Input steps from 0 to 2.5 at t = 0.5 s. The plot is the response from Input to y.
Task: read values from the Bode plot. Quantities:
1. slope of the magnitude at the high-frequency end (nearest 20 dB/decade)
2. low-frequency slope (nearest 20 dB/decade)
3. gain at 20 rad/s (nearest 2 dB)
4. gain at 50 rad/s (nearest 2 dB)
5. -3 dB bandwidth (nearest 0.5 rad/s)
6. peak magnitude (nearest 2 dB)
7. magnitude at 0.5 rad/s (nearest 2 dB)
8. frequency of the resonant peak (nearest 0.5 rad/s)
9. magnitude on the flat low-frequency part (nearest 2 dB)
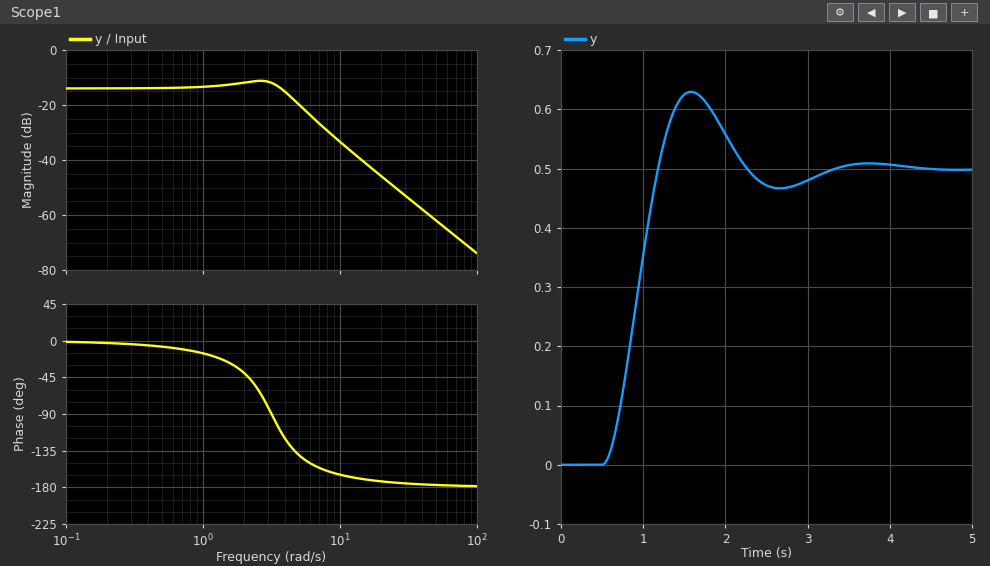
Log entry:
-40 dB/decade
0 dB/decade
-46 dB
-62 dB
4.5 rad/s
-12 dB
-14 dB
2.5 rad/s
-14 dB
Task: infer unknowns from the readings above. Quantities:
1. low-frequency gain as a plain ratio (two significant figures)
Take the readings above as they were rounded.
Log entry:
0.20
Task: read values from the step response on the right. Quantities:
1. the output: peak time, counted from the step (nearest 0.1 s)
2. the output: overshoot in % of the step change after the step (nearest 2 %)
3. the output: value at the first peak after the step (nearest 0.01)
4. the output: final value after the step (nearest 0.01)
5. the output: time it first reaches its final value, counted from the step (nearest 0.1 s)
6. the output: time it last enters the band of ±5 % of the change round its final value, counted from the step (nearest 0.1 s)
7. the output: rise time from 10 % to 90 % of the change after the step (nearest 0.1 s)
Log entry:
1.1 s
26 %
0.63
0.50
0.7 s
2.4 s
0.5 s
